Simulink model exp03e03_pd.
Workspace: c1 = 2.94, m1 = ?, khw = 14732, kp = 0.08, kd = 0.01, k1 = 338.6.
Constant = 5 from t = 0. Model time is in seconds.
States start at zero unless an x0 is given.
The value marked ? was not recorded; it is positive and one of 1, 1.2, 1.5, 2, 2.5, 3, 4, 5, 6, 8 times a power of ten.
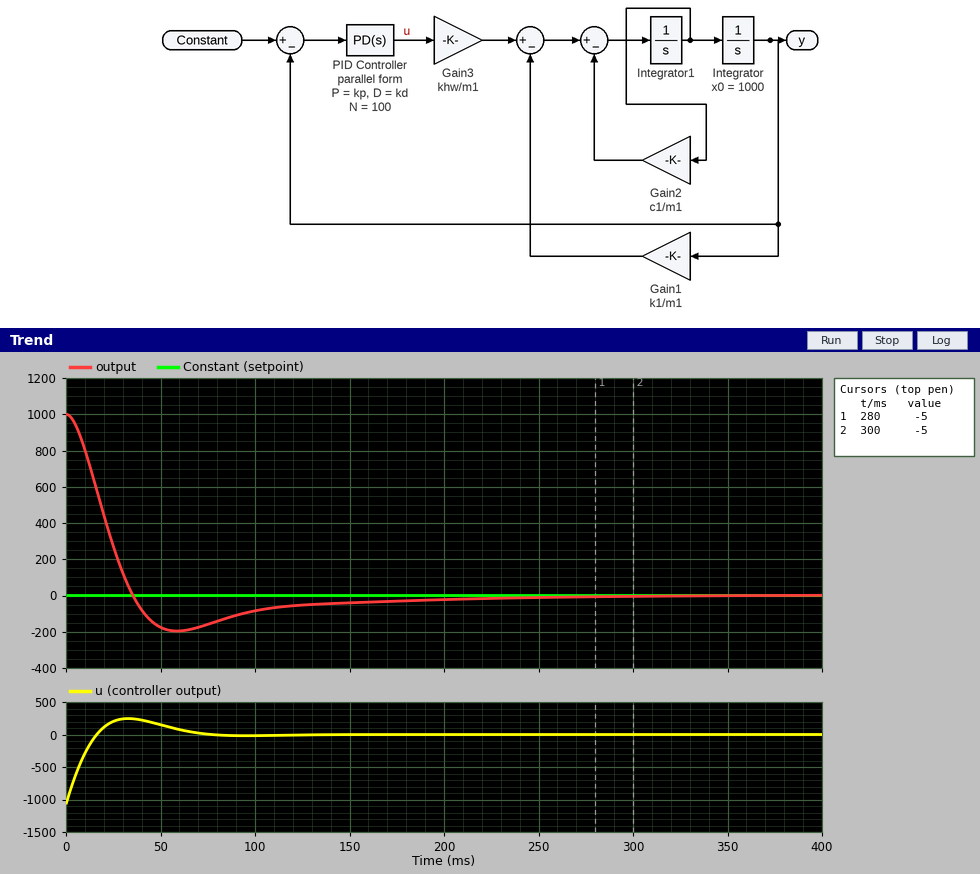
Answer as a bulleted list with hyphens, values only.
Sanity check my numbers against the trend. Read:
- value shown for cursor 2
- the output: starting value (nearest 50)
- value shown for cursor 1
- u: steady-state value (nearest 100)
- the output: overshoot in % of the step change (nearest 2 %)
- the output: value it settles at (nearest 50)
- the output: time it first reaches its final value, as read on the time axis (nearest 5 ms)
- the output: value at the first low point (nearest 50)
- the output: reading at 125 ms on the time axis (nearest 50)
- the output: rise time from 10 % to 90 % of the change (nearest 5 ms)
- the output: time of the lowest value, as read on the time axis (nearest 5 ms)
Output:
- -5
- 1000
- -5
- 0
- 20 %
- 0
- 35 ms
- -200
- -50
- 25 ms
- 60 ms
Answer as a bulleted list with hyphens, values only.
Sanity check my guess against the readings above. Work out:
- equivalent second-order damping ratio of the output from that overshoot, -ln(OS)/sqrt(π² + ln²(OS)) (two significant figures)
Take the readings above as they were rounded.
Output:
- 0.46
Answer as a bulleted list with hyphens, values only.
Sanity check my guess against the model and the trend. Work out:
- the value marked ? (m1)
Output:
- 3
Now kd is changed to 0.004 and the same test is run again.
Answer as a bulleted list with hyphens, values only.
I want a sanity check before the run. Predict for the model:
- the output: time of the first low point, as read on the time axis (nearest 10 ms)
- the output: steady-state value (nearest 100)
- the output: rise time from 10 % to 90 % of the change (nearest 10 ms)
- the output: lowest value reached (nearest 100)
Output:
- 100 ms
- 0
- 40 ms
- -400
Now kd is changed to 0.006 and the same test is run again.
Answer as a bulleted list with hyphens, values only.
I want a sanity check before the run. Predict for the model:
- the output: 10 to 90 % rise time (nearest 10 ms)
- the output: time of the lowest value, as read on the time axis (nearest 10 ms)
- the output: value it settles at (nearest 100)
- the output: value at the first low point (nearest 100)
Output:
- 30 ms
- 80 ms
- 0
- -300
